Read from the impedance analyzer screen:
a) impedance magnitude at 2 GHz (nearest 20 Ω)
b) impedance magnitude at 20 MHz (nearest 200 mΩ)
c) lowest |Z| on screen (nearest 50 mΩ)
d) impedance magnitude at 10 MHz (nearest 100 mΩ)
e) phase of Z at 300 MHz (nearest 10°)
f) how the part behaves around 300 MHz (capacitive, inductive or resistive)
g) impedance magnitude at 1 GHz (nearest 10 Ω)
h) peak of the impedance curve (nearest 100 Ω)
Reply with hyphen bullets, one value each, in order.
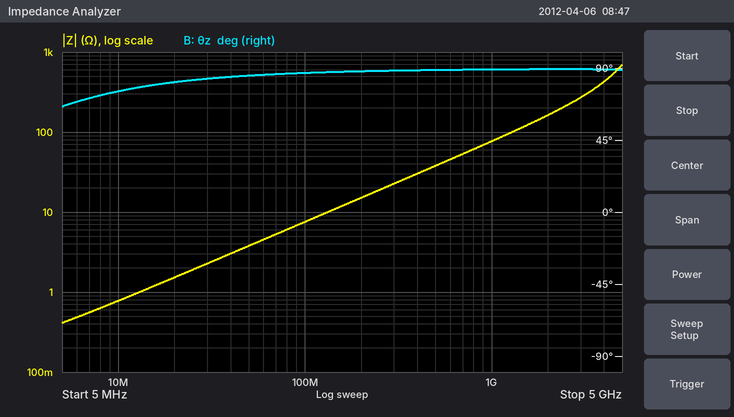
- 160 Ω
- 1.6 Ω
- 400 mΩ
- 800 mΩ
- 90°
- inductive
- 80 Ω
- 700 Ω
